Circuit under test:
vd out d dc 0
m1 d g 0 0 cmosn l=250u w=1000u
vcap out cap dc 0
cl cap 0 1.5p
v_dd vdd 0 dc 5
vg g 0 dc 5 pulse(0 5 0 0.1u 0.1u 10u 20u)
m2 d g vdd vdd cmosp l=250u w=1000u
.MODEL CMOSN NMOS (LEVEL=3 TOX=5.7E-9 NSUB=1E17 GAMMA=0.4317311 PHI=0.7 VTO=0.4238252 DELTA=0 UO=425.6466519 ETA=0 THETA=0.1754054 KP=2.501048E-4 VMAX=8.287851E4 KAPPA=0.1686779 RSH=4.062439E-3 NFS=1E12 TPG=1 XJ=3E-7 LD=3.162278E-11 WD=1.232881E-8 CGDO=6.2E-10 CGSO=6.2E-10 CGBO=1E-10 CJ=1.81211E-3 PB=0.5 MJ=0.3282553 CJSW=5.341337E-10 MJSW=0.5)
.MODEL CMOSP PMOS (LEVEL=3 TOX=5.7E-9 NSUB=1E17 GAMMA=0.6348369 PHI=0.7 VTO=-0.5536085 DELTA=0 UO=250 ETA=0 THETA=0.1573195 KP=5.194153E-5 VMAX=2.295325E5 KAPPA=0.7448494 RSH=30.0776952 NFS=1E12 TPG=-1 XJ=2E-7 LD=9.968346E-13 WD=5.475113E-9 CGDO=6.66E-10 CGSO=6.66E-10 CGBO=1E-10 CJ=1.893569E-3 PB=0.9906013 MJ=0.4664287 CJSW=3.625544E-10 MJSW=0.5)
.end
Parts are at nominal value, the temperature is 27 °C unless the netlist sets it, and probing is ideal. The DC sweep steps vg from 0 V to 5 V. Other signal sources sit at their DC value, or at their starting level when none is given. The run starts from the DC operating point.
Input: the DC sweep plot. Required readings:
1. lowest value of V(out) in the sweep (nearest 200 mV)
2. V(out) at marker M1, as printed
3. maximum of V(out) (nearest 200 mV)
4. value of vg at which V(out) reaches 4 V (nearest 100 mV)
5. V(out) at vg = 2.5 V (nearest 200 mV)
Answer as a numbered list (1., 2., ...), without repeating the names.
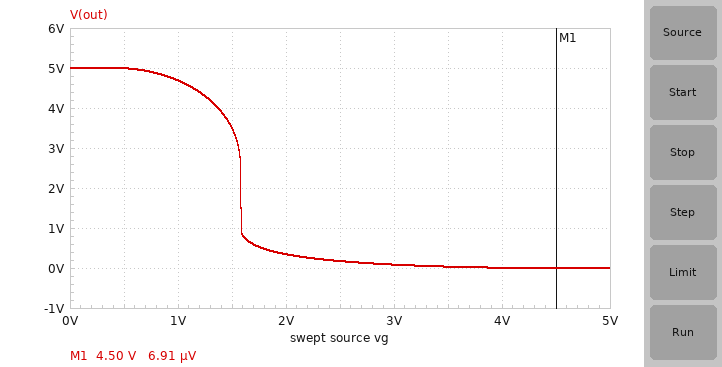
1. 0 V
2. 6.91 µV
3. 5.0 V
4. 1.4 V
5. 200 mV
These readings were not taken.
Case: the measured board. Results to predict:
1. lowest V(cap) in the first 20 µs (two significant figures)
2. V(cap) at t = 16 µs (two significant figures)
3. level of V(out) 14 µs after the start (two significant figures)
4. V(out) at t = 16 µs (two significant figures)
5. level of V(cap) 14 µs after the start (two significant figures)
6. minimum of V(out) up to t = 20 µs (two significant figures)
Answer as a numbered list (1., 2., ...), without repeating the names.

1. -760 mV
2. 4.9 V
3. 4.7 V
4. 4.9 V
5. 4.7 V
6. -760 mV
